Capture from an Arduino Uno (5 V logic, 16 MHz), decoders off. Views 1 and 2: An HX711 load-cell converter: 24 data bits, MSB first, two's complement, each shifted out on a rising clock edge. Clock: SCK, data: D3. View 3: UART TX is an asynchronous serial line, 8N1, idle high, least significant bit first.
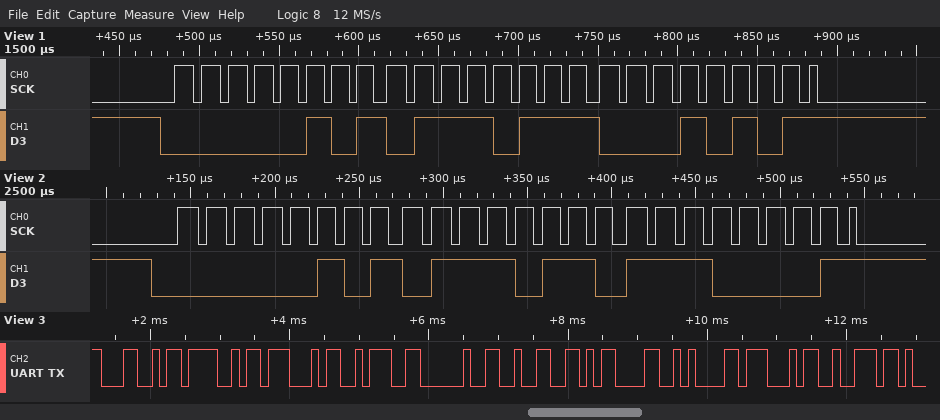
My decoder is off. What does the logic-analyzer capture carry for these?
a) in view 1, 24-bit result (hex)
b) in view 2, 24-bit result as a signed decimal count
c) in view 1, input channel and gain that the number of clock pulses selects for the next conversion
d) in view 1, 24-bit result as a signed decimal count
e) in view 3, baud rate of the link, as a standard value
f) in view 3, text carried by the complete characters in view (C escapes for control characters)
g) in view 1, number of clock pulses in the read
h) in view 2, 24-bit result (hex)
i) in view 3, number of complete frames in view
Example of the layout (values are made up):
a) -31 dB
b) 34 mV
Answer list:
a) 0x057715
b) 358113
c) channel A, gain 128
d) 358165
e) 9600 baud
f) "LOG: 2\r\nGr"
g) 25
h) 0x0576E1
i) 10
